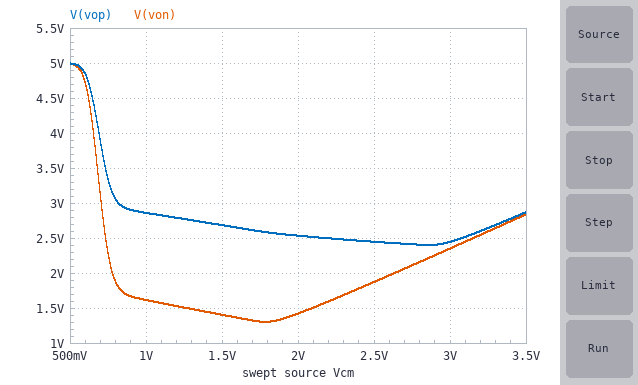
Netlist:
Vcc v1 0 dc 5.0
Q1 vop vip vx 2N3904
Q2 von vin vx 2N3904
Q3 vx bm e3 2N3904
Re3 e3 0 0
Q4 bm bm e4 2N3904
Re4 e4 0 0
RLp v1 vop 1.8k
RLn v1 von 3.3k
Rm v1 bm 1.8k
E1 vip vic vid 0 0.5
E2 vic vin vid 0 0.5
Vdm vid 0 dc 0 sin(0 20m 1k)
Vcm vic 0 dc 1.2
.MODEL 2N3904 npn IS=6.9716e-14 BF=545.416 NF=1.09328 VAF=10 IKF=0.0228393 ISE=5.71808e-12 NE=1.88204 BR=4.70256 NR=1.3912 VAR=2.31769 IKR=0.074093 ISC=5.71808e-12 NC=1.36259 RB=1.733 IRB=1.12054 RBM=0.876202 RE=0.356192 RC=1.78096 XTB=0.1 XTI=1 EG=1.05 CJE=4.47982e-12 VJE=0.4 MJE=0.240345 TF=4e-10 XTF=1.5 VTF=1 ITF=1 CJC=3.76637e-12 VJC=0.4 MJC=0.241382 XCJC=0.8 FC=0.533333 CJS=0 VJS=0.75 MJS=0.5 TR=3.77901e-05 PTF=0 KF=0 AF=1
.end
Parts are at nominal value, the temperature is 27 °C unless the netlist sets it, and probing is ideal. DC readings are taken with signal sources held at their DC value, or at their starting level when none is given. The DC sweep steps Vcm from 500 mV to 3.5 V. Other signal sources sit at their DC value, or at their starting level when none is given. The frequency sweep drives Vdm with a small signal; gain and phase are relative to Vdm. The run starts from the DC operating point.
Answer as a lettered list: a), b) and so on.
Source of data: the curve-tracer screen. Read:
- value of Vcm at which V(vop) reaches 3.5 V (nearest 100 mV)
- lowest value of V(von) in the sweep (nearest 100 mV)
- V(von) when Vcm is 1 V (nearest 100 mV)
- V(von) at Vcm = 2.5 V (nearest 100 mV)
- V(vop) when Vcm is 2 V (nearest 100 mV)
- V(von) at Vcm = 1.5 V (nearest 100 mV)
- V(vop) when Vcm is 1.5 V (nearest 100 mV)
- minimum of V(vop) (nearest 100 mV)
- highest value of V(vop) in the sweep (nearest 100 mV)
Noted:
a) 700 mV
b) 1.3 V
c) 1.6 V
d) 1.9 V
e) 2.5 V
f) 1.4 V
g) 2.7 V
h) 2.4 V
i) 5.0 V
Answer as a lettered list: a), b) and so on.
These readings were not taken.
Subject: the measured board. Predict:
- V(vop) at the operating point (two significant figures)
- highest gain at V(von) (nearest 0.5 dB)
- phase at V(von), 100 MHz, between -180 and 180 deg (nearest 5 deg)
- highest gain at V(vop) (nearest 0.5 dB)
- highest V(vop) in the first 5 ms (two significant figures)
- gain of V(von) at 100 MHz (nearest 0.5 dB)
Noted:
a) 2.8 V
b) 33.0 dB
c) -85 deg
d) 28.0 dB
e) 3.3 V
f) 18.5 dB
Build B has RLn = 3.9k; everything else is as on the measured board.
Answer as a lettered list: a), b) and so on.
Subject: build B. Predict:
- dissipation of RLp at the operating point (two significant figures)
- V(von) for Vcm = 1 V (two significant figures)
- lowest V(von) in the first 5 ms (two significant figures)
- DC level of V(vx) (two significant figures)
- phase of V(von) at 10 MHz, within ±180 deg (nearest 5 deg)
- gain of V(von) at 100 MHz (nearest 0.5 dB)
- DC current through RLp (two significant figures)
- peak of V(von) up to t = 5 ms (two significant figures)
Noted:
a) 2.9 mW
b) 1.1 V
c) 600 mV
d) 530 mV
e) -40 deg
f) 16.0 dB
g) 1.3 mA
h) 2.0 V
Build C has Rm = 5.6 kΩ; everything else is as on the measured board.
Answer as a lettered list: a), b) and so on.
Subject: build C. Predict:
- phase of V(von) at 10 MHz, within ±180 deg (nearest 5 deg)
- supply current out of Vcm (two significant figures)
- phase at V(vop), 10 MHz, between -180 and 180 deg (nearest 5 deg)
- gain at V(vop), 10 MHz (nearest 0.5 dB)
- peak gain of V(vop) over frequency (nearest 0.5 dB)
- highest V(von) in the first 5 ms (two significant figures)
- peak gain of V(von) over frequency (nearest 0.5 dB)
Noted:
a) -25 deg
b) 6.5 µA
c) 165 deg
d) 20.0 dB
e) 20.5 dB
f) 4.2 V
g) 25.5 dB
